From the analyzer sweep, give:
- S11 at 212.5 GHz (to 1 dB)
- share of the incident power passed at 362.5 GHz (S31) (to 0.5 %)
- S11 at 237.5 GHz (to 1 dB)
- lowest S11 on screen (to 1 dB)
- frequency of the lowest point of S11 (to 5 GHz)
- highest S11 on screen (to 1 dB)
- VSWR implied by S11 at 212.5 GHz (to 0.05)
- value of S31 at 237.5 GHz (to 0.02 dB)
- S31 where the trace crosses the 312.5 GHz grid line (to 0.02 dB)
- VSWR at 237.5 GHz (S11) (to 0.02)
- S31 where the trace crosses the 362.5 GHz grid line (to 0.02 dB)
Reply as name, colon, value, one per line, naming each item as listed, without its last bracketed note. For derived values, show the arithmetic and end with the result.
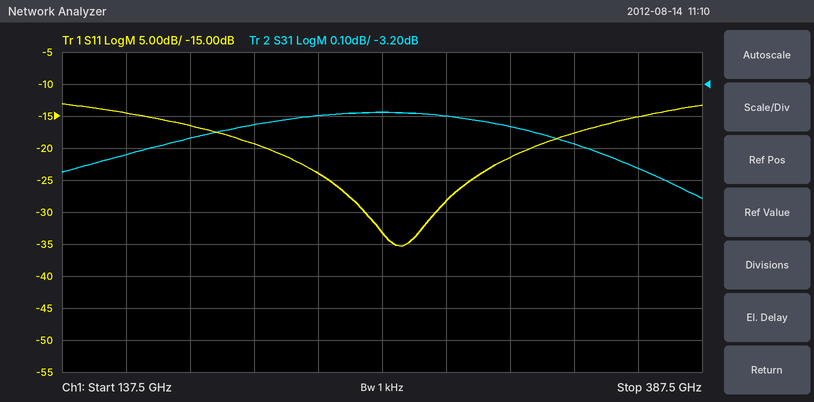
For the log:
S11 at 212.5 GHz: -19 dB
share of the incident power passed at 362.5 GHz (S31): 10^(-3.46/10) ≈ 45.1 %, so 45.0 % to the nearest 0.5 %
S11 at 237.5 GHz: -24 dB
lowest S11 on screen: -35 dB
frequency of the lowest point of S11: 270 GHz
highest S11 on screen: -13 dB
VSWR implied by S11 at 212.5 GHz: |Γ| = 10^(-19/20) = 0.1122; VSWR = (1 + 0.1122)/(1 − 0.1122) ≈ 1.25
value of S31 at 237.5 GHz: -3.30 dB
S31 where the trace crosses the 312.5 GHz grid line: -3.34 dB
VSWR at 237.5 GHz (S11): |Γ| = 10^(-24/20) = 0.0631; VSWR = (1 + 0.0631)/(1 − 0.0631) ≈ 1.13, so 1.14 to the nearest 0.02
S31 where the trace crosses the 362.5 GHz grid line: -3.46 dB
